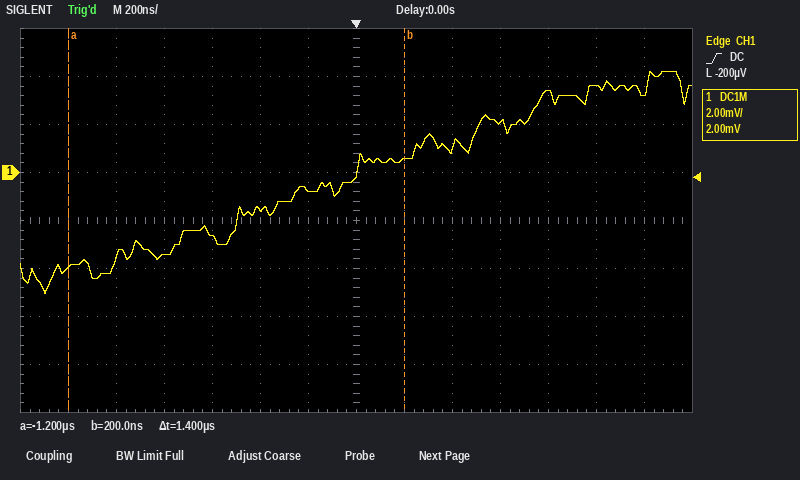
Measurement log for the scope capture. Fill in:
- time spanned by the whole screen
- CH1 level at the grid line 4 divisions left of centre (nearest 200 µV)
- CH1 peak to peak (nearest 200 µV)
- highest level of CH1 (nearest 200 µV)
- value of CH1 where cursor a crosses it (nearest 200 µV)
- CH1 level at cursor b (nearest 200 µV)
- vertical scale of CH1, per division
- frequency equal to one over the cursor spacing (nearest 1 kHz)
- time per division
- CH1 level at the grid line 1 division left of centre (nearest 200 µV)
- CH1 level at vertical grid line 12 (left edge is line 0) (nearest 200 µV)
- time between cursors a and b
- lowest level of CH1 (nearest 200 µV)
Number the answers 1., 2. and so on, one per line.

1. 2.8 µs
2. -3.4 mV
3. 9.2 mV
4. 4.2 mV
5. -4.0 mV
6. 600 µV
7. 2 mV
8. 714 kHz
9. 200 ns
10. -800 µV
11. 3.6 mV
12. 1.4 µs
13. -5.0 mV
